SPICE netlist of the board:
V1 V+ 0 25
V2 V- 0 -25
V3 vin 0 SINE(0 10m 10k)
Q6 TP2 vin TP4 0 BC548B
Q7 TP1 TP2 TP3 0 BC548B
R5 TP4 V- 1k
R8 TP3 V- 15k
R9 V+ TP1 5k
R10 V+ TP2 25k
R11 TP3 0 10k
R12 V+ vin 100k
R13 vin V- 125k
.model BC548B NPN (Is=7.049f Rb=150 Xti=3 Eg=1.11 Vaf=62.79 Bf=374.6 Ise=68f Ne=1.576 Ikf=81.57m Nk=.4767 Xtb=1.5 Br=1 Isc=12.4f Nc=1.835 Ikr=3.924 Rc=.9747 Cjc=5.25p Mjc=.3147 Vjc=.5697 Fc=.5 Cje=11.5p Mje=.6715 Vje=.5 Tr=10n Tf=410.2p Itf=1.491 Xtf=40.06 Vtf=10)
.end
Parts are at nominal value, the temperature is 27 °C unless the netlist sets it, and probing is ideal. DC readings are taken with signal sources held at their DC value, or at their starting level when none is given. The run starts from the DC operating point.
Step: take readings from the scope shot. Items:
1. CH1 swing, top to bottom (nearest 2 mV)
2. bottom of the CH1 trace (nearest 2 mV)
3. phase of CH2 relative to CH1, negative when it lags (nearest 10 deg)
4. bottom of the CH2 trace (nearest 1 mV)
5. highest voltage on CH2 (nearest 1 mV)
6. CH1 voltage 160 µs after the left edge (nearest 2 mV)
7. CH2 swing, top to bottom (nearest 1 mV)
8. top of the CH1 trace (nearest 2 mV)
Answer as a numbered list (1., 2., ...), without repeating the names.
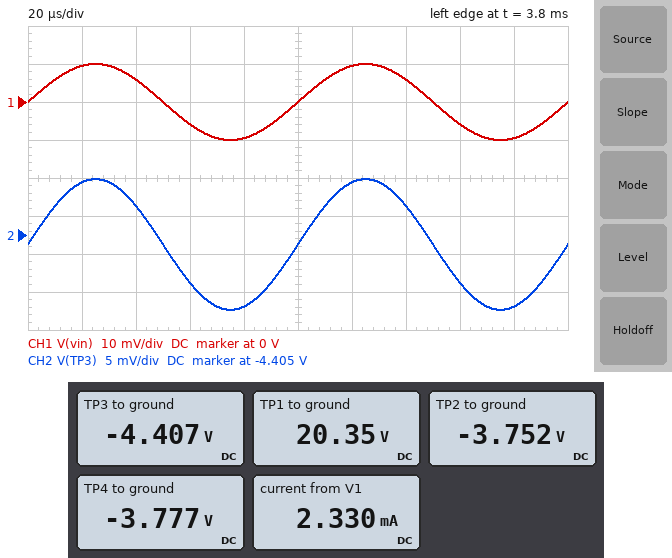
1. 20 mV
2. -10 mV
3. 0 deg
4. -4.415 V
5. -4.398 V
6. -6 mV
7. 17 mV
8. 10 mV
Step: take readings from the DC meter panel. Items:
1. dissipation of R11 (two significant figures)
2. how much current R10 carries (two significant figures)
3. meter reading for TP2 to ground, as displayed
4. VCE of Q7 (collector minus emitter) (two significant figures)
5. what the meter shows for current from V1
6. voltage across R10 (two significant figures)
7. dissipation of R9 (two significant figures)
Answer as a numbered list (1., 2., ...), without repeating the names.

1. 1.9 mW
2. 1.2 mA
3. -3.752 V
4. 25 V
5. 2.330 mA
6. 29 V
7. 4.3 mW
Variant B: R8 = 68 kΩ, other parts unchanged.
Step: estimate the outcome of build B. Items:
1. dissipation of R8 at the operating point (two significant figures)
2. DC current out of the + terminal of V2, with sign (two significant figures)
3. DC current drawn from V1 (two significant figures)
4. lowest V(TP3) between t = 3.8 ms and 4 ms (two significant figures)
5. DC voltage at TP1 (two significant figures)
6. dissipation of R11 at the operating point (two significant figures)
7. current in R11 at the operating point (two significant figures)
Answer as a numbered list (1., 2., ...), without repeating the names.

1. 7.0 mW
2. -22 mA
3. 1.4 mA
4. -3.2 V
5. 25 V
6. 1.0 mW
7. 320 µA
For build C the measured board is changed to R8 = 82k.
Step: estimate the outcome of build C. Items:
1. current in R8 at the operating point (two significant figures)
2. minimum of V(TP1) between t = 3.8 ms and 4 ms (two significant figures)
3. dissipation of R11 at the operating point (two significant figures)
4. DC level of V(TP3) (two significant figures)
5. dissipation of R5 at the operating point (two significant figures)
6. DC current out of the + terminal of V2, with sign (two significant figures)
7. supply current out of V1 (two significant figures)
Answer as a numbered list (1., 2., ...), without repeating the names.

1. 270 µA
2. 25 V
3. 740 µW
4. -2.7 V
5. 450 mW
6. -22 mA
7. 1.4 mA
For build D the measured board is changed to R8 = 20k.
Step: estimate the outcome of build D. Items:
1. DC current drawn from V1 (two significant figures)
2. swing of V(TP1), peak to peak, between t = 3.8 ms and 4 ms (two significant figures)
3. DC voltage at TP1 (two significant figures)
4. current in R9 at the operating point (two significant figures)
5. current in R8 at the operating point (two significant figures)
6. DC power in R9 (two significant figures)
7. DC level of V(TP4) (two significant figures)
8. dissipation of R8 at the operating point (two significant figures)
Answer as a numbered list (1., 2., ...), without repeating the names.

1. 2.0 mA
2. 13 mV
3. 22 V
4. 590 µA
5. 1.0 mA
6. 1.7 mW
7. -3.8 V
8. 21 mW
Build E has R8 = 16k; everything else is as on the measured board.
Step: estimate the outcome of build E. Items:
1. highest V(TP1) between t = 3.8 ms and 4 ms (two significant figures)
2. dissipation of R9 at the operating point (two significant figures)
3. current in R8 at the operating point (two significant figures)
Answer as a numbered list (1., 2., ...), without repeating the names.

1. 21 V
2. 3.6 mW
3. 1.3 mA
